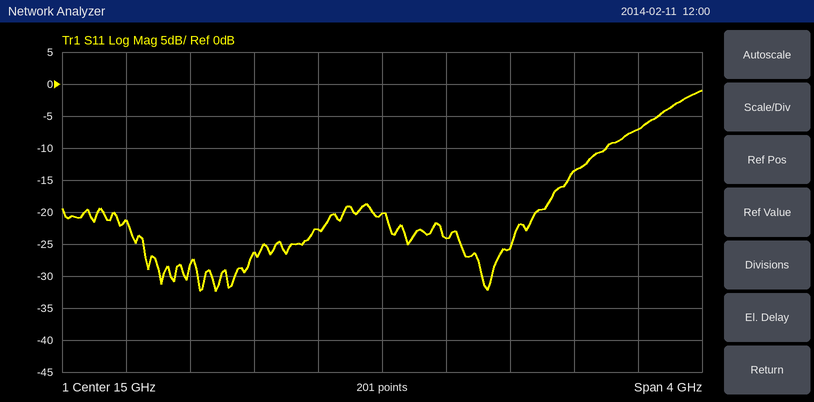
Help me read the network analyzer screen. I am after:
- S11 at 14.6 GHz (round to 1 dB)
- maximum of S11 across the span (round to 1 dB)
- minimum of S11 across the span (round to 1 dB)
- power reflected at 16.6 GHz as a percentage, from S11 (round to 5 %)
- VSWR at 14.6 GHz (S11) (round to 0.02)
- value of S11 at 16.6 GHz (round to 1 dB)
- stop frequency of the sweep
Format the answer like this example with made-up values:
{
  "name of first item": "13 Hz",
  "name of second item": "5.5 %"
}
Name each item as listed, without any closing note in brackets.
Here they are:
{
  "S11 at 14.6 GHz": "-23 dB",
  "maximum of S11 across the span": "-1 dB",
  "minimum of S11 across the span": "-32 dB",
  "power reflected at 16.6 GHz as a percentage, from S11": "20 %",
  "VSWR at 14.6 GHz (S11)": "1.16",
  "value of S11 at 16.6 GHz": "-7 dB",
  "stop frequency of the sweep": "17 GHz"
}
